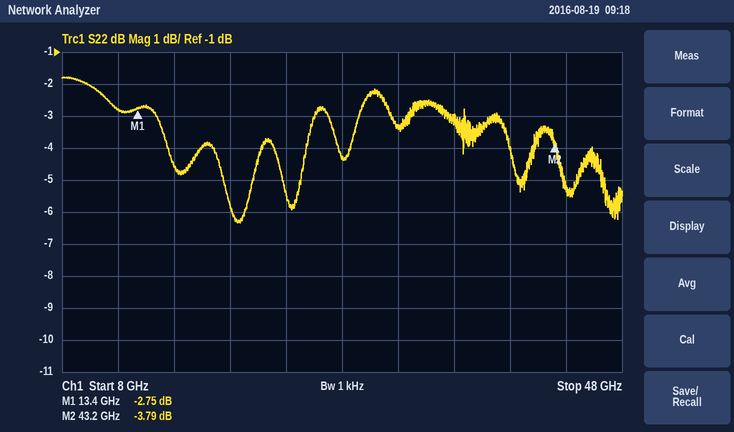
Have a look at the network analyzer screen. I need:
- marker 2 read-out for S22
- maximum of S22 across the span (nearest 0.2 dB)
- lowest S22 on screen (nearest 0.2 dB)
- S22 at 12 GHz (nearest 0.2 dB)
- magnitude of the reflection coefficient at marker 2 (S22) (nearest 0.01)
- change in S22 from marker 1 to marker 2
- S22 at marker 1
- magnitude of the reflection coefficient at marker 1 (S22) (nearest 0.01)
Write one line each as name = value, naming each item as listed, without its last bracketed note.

marker 2 read-out for S22 = -3.79 dB
maximum of S22 across the span = -1.8 dB
lowest S22 on screen = -6.4 dB
S22 at 12 GHz = -2.8 dB
magnitude of the reflection coefficient at marker 2 (S22) = 0.65
change in S22 from marker 1 to marker 2 = -1.04 dB
S22 at marker 1 = -2.75 dB
magnitude of the reflection coefficient at marker 1 (S22) = 0.73
